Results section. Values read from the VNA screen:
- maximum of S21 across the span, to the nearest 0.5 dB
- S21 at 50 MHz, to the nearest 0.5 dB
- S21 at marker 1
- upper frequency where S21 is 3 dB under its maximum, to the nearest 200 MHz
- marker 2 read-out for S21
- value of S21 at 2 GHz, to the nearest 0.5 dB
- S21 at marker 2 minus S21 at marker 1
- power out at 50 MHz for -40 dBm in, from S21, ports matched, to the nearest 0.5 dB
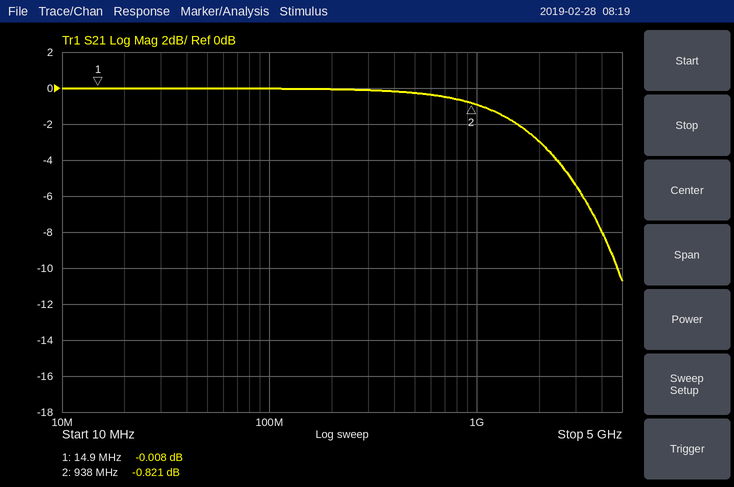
0.0 dB
0.0 dB
-0.008 dB
2.0 GHz
-0.821 dB
-3.0 dB
-0.813 dB
-40.0 dBm
